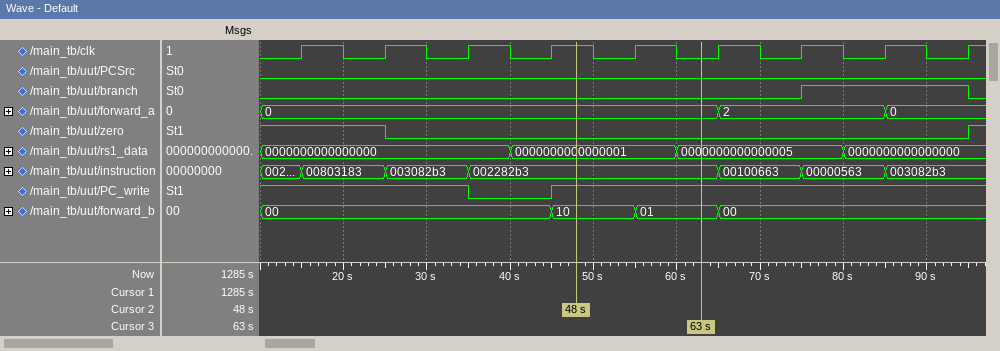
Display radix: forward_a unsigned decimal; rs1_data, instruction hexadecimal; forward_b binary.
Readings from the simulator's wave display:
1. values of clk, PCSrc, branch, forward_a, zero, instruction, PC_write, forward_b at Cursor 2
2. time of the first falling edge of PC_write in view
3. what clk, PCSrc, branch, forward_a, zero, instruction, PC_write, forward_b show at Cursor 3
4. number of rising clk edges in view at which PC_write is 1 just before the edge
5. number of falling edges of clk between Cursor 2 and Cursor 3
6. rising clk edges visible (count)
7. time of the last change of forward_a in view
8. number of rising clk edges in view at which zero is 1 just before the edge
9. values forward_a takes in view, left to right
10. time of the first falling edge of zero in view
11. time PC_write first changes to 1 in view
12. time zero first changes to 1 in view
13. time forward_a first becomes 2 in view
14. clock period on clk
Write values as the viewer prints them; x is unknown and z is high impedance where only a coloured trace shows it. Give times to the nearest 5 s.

clk=1, PCSrc=0, branch=0, forward_a=0, zero=0, instruction=002282b3, PC_write=1, forward_b=10
35 s
clk=0, PCSrc=0, branch=0, forward_a=0, zero=0, instruction=002282b3, PC_write=1, forward_b=01
8
2
9
85 s
2
0, 2, 0
25 s
45 s
95 s
65 s
10 s
